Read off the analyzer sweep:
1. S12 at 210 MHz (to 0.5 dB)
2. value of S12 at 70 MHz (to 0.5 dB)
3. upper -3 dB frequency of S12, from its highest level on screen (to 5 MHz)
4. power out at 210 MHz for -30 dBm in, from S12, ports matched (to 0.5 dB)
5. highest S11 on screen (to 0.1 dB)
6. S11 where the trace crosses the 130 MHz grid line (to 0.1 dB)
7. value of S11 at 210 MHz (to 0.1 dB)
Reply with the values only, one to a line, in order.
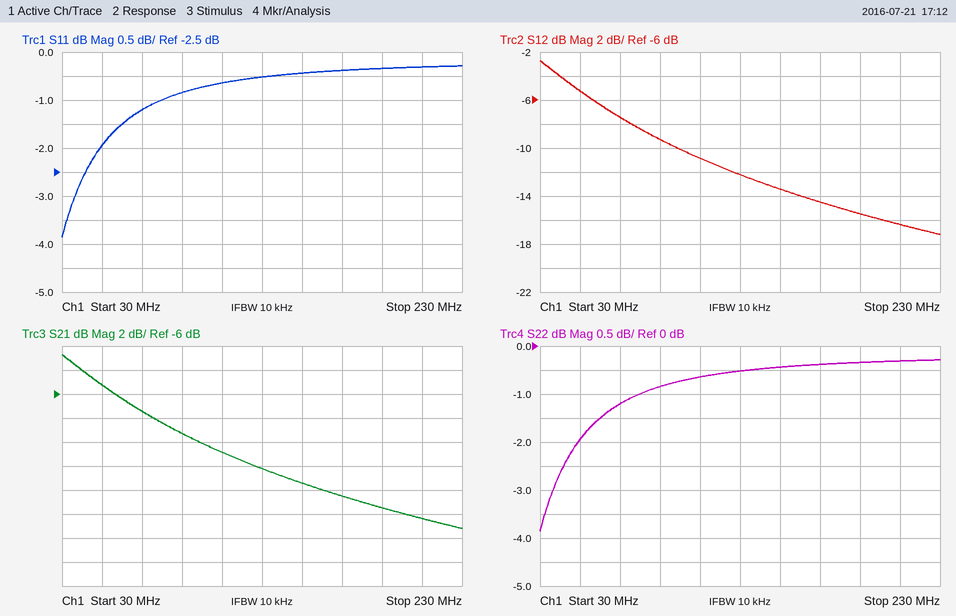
-16.5 dB
-7.5 dB
55 MHz
-46.5 dBm
-0.3 dB
-0.5 dB
-0.3 dB
